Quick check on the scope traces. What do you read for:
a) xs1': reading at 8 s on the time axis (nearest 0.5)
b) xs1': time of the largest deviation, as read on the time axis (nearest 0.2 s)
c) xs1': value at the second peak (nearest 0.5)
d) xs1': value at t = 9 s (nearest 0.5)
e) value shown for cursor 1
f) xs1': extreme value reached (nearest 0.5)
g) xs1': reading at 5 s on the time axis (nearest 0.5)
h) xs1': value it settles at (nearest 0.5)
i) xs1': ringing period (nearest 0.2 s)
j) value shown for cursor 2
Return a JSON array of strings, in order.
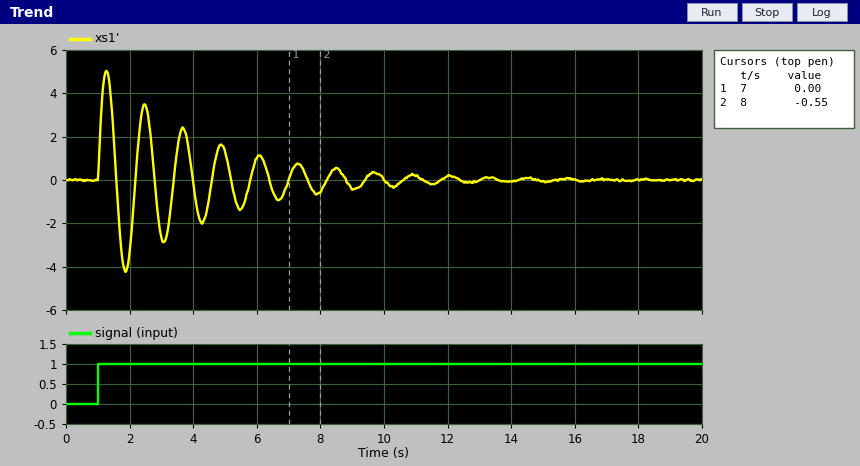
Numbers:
["-0.5", "1.2 s", "3.5", "-0.5", "0.00", "5.0", "1.5", "0.0", "1.2 s", "-0.55"]
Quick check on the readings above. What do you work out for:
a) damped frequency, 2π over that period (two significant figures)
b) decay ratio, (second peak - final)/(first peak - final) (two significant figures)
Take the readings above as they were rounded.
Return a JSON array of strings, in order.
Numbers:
["5.2 rad/s", "0.70"]
